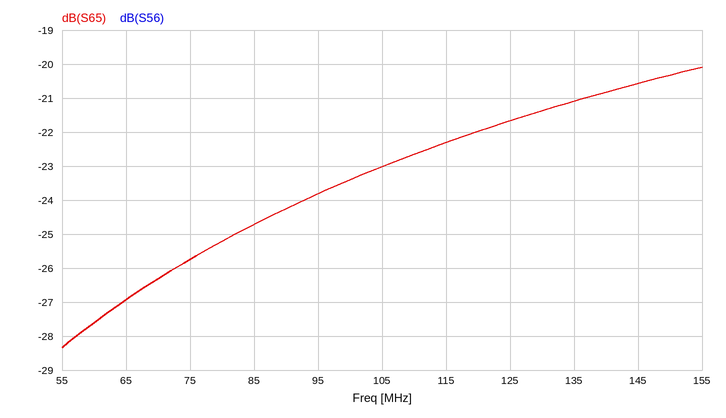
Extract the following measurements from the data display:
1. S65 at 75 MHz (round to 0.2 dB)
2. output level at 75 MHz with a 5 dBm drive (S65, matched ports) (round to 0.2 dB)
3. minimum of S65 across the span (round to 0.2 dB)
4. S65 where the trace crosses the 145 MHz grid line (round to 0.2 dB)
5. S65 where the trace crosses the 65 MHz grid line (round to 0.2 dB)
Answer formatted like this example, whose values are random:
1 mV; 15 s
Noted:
-25.8 dB; -20.8 dBm; -28.4 dB; -20.6 dB; -27.0 dB
